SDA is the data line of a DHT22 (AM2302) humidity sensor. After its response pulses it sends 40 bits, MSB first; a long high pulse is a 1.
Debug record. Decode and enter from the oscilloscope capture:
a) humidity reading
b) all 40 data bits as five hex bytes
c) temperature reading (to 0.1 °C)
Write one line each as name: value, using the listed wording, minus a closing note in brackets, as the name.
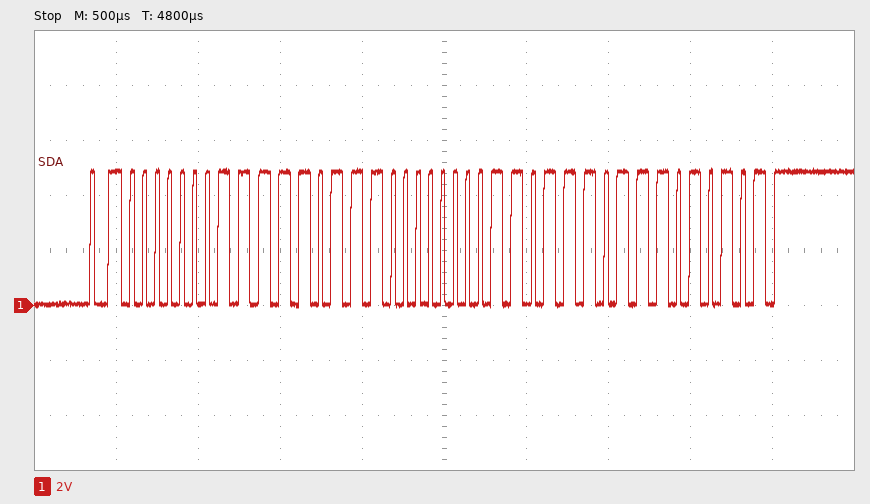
humidity reading: 50.3 %
all 40 data bits as five hex bytes: 01 F7 00 DD D5
temperature reading: 22.1 °C
